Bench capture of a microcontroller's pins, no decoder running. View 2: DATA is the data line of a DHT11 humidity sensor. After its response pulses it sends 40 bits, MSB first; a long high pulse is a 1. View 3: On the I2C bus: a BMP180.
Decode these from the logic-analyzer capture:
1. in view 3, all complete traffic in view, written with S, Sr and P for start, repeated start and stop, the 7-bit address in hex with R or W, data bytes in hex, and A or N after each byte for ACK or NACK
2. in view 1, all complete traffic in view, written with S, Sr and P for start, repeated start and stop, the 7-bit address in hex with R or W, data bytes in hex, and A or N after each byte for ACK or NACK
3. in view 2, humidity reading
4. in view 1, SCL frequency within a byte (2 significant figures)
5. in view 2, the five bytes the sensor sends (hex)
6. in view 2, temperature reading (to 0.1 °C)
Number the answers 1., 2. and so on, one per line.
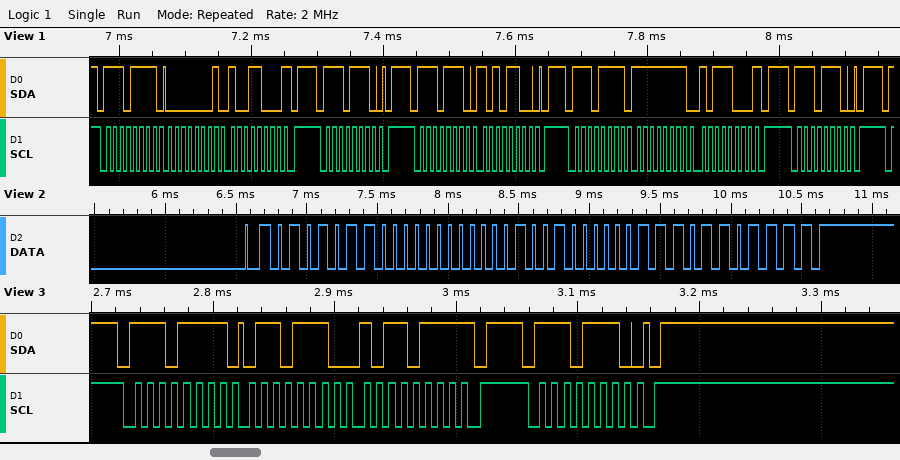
1. S 77R A 6E A B7 N P S 77W A P
2. S 77R A 01 A 98 N P S 77W A P S 77W A AC A P S 77R A FF A B8 N P S 77W A P
3. 86 %
4. 100 kHz
5. 56 00 12 07 6F
6. 18.7 °C
